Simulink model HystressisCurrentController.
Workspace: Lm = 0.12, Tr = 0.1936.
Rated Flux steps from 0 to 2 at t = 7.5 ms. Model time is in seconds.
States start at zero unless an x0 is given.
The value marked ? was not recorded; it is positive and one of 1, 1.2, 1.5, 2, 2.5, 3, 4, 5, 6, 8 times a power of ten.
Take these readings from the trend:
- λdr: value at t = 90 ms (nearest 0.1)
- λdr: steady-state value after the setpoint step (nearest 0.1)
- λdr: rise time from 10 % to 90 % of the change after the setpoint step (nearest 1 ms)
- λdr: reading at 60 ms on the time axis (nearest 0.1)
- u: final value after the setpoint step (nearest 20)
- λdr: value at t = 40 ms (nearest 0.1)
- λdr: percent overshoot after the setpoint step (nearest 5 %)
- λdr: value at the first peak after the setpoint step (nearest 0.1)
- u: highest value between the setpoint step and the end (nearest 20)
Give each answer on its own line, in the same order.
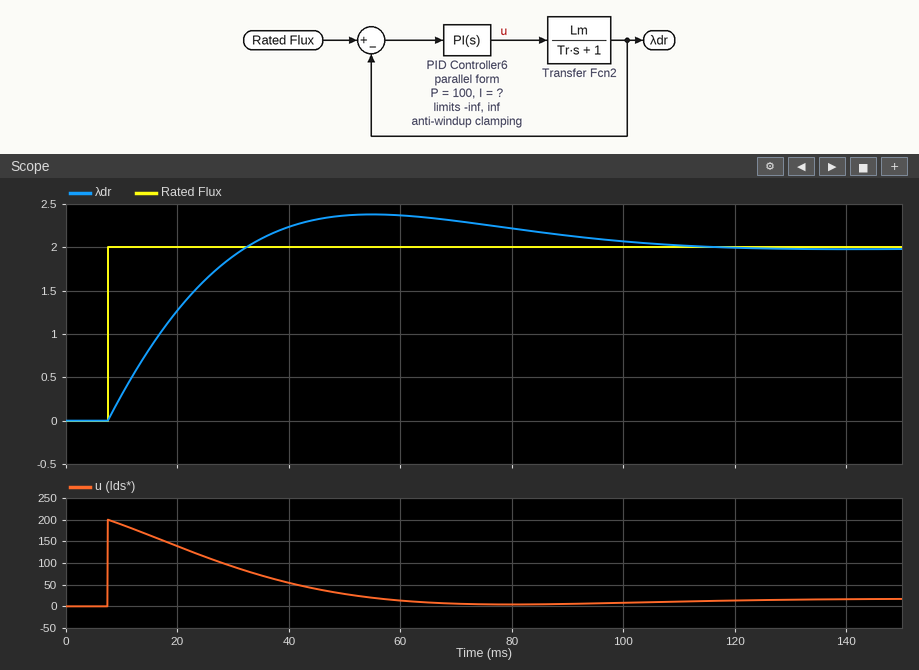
2.1
2.0
19 ms
2.4
20
2.2
20 %
2.4
200
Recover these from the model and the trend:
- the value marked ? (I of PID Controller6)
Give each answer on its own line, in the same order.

4000
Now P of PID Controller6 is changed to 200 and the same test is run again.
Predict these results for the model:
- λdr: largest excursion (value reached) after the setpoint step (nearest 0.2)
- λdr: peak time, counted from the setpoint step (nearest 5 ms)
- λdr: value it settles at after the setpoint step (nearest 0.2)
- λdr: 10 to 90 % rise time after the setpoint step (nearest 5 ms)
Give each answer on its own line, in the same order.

2.2
40 ms
2.0
15 ms
